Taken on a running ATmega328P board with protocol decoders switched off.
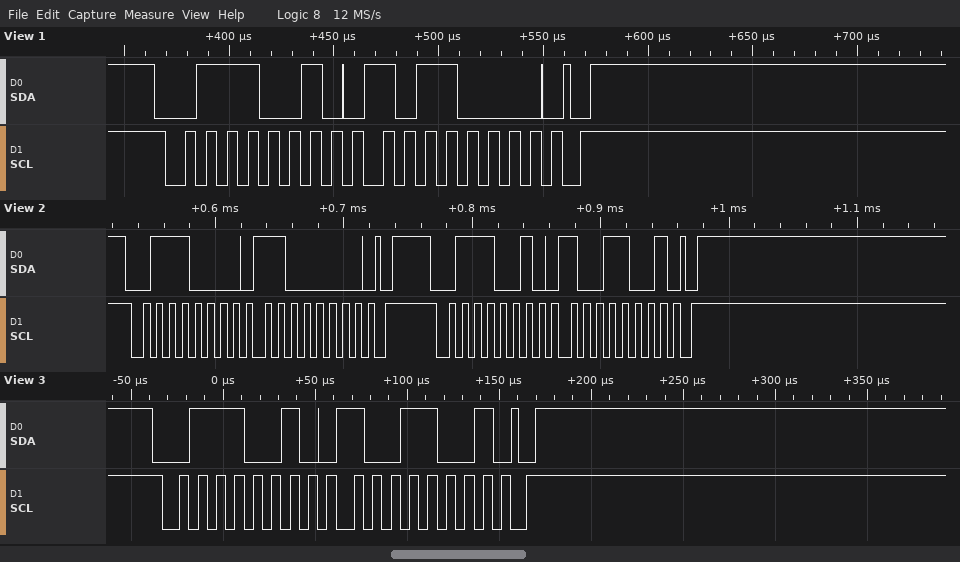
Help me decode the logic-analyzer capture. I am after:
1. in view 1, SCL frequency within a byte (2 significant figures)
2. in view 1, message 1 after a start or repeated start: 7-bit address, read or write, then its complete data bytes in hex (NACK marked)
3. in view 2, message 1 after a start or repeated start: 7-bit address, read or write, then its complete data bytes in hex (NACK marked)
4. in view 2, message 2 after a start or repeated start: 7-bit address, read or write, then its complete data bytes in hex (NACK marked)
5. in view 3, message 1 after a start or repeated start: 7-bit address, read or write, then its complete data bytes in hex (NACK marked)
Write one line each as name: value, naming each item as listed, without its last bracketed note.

in view 1, SCL frequency within a byte: 100 kHz
in view 1, message 1 after a start or repeated start: 7-bit address, read or write, then its complete data bytes in hex: 0x39 write: B0
in view 2, message 1 after a start or repeated start: 7-bit address, read or write, then its complete data bytes in hex: 0x38 write: C0
in view 2, message 2 after a start or repeated start: 7-bit address, read or write, then its complete data bytes in hex: 0x39 write: 99
in view 3, message 1 after a start or repeated start: 7-bit address, read or write, then its complete data bytes in hex: 0x39 write: 99
